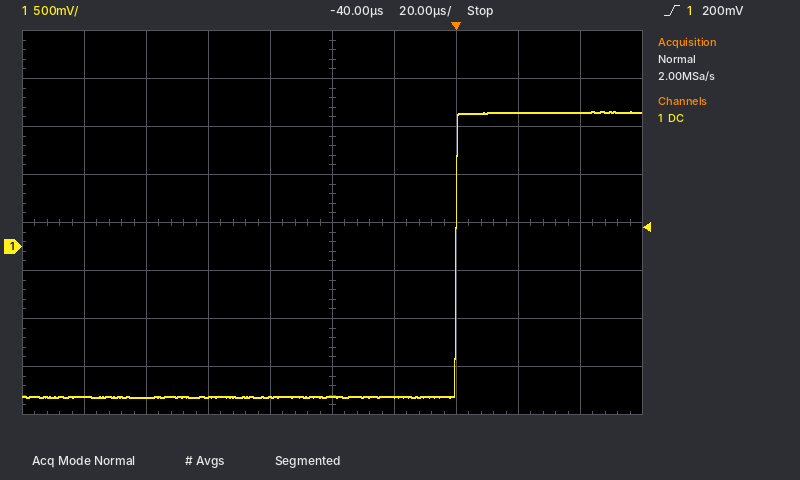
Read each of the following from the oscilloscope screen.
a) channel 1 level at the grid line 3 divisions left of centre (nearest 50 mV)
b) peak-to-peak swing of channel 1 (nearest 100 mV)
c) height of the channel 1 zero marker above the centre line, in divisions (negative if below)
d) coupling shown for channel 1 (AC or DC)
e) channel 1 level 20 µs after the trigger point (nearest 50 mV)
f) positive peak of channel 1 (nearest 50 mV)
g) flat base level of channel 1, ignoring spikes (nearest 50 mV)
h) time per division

-1.55 V
3.00 V
-0.5 div
DC
1.40 V
1.40 V
-1.55 V
20 µs
